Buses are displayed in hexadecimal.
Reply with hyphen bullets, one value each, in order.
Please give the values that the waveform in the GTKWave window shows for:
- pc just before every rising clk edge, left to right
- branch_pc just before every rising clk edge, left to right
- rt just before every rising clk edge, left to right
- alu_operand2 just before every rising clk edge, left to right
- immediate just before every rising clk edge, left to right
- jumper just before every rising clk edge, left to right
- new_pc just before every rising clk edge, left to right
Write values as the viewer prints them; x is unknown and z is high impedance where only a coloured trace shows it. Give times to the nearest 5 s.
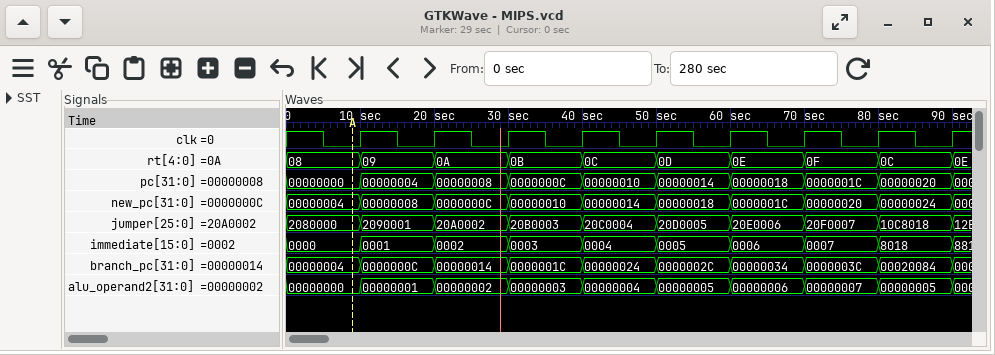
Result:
- 00000000, 00000004, 00000008, 0000000C, 00000010, 00000014, 00000018, 0000001C, 00000020
- 00000004, 0000000C, 00000014, 0000001C, 00000024, 0000002C, 00000034, 0000003C, 00020084
- 08, 09, 0A, 0B, 0C, 0D, 0E, 0F, 0C
- 00000000, 00000001, 00000002, 00000003, 00000004, 00000005, 00000006, 00000007, 00000005
- 0000, 0001, 0002, 0003, 0004, 0005, 0006, 0007, 8018
- 2080000, 2090001, 20A0002, 20B0003, 20C0004, 20D0005, 20E0006, 20F0007, 10C8018
- 00000004, 00000008, 0000000C, 00000010, 00000014, 00000018, 0000001C, 00000020, 00000024
